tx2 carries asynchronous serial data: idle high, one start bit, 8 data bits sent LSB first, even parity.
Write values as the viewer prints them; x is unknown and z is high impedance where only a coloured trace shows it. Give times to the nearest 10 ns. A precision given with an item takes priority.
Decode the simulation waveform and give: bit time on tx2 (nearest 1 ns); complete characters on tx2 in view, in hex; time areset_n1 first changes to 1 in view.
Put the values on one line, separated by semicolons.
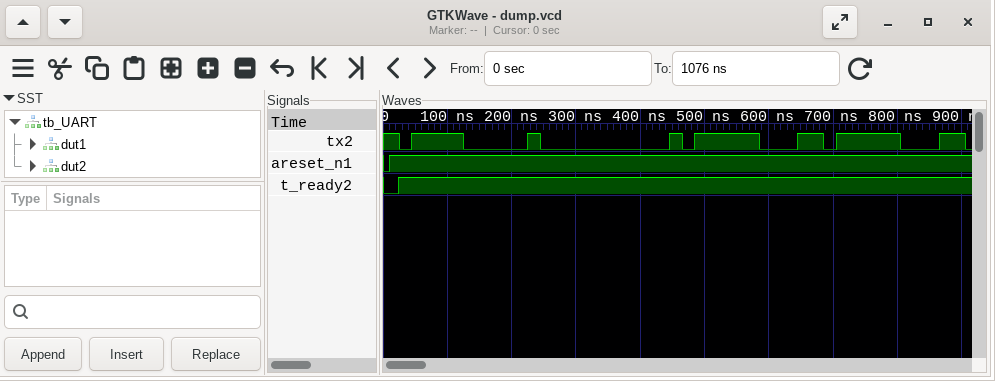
20 ns; 0F, 00, 1F, 1F; 10 ns
